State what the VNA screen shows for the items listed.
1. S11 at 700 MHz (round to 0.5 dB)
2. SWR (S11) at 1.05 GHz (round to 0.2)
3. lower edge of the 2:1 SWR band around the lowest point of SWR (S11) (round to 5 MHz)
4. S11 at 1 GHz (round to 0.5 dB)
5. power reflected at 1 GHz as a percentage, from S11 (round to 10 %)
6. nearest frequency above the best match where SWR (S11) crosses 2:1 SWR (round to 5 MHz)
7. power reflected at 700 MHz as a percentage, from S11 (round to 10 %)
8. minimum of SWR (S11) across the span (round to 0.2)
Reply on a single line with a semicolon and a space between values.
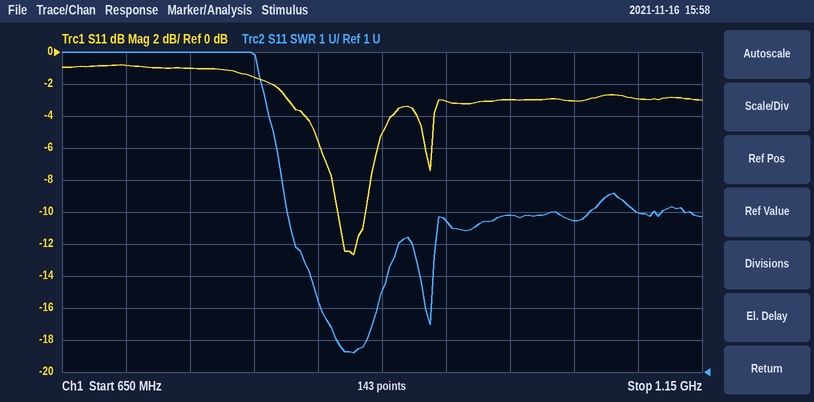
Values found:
-1.0 dB; 5.8; 865 MHz; -3.0 dB; 50 %; 890 MHz; 80 %; 1.6
